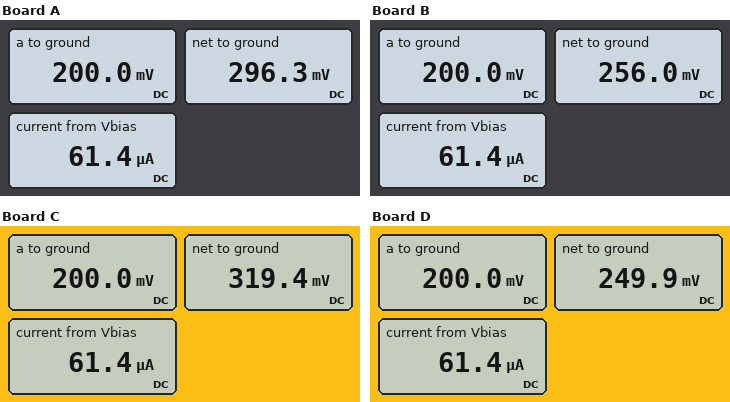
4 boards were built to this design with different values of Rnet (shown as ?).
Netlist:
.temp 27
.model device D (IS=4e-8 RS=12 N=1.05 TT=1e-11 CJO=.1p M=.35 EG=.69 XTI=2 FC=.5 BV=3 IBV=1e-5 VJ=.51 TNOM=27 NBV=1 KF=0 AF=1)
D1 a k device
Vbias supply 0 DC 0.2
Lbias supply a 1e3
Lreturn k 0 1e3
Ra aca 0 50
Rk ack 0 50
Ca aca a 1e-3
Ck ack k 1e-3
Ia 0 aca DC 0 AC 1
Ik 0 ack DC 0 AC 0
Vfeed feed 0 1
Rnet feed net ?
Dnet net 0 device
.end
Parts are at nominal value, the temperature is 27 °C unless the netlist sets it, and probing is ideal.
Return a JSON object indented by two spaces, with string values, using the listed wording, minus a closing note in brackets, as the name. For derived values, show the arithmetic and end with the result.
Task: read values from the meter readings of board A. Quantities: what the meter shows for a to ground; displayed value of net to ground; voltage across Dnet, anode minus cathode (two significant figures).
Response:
{
  "what the meter shows for a to ground": "200.0 mV",
  "displayed value of net to ground": "296.3 mV",
  "voltage across Dnet, anode minus cathode": "296.3 mV = 300 mV"
}
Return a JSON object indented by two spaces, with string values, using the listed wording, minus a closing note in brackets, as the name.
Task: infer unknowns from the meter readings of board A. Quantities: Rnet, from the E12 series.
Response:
{
  "Rnet, from the E12 series": "560 Ω"
}
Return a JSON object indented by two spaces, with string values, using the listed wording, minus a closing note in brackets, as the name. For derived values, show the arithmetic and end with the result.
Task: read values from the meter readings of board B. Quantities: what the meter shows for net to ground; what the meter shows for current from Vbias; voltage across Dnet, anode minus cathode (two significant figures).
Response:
{
  "what the meter shows for net to ground": "256.0 mV",
  "what the meter shows for current from Vbias": "61.4 µA",
  "voltage across Dnet, anode minus cathode": "256 mV = 260 mV"
}
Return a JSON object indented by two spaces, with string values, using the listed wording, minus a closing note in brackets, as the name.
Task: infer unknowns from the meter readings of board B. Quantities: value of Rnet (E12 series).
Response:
{
  "value of Rnet": "1.8 kΩ"
}
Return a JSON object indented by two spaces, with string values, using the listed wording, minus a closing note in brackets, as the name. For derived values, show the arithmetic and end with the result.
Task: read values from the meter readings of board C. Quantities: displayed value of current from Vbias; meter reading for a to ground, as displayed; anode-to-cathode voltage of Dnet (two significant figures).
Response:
{
  "displayed value of current from Vbias": "61.4 µA",
  "meter reading for a to ground, as displayed": "200.0 mV",
  "anode-to-cathode voltage of Dnet": "319.4 mV = 320 mV"
}
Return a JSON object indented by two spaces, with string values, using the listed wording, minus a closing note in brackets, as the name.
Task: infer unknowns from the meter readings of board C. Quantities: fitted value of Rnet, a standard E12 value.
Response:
{
  "fitted value of Rnet, a standard E12 value": "330 Ω"
}
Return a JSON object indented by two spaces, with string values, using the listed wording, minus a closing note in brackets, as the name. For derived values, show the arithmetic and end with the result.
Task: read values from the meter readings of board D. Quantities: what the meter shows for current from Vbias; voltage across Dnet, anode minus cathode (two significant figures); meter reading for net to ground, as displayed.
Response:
{
  "what the meter shows for current from Vbias": "61.4 µA",
  "voltage across Dnet, anode minus cathode": "249.9 mV = 250 mV",
  "meter reading for net to ground, as displayed": "249.9 mV"
}
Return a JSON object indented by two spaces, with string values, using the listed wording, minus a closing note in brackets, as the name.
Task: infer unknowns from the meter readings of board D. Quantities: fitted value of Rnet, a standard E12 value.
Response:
{
  "fitted value of Rnet, a standard E12 value": "2.2 kΩ"
}
